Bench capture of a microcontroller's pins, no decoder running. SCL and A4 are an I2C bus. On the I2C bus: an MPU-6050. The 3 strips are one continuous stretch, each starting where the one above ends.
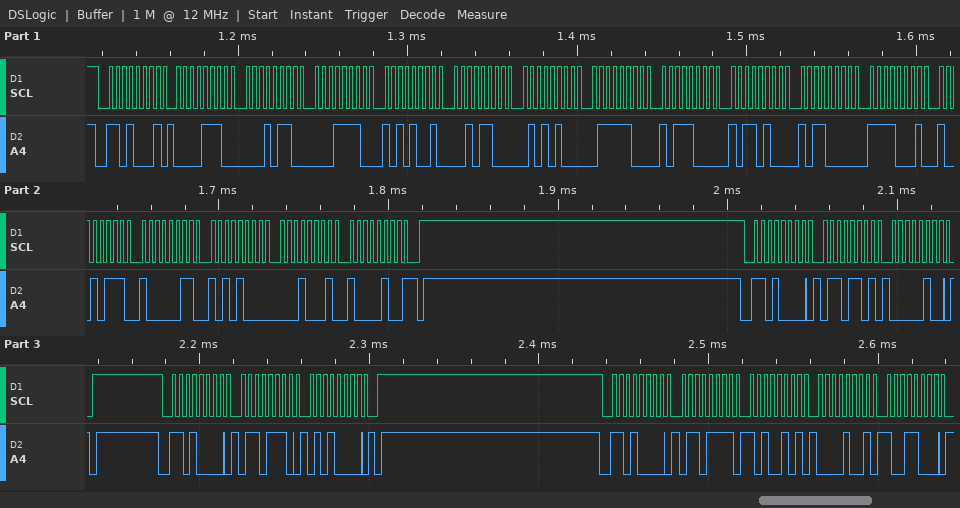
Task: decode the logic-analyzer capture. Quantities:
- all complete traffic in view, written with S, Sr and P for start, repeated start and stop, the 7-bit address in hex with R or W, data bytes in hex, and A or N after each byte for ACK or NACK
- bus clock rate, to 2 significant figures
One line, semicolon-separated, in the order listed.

S 68R A 0E A 16 A 1E A A9 A 2C A 54 A 7C A B8 A B4 A B0 A F1 A 97 A 83 A A8 A 11 A 84 N P S 68W A 6D A 04 A P S 68W A 6E A 50 A P S 68W A 6F A A5 A 09 A 98 A; 250 kHz
